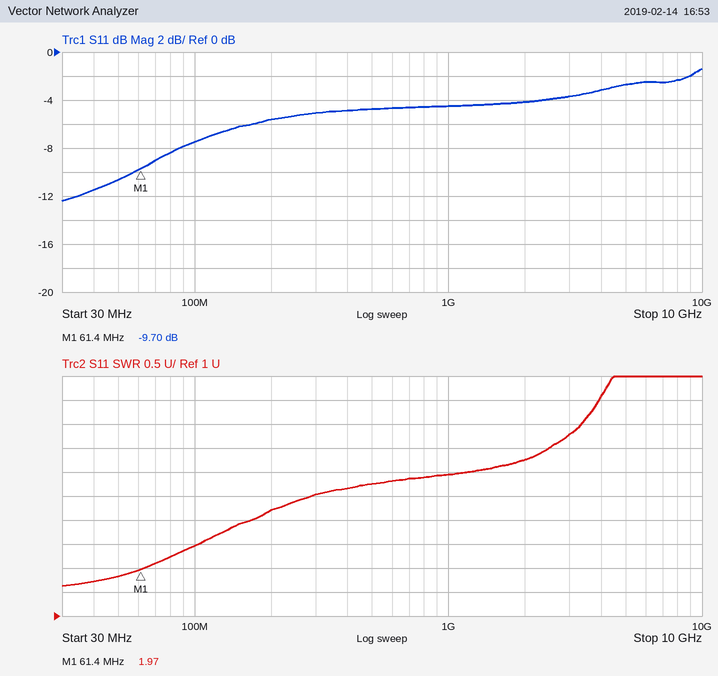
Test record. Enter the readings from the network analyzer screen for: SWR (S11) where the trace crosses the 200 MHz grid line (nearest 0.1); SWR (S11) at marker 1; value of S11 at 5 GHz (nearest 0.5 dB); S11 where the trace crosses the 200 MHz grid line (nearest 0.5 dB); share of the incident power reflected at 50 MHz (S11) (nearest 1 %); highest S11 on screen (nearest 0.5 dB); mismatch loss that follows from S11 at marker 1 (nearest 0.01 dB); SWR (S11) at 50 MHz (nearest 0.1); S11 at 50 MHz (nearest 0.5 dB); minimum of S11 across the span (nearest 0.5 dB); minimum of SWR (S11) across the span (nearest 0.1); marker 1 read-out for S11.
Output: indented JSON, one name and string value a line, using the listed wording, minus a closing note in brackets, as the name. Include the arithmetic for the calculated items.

{
  "SWR (S11) where the trace crosses the 200 MHz grid line": "3.2",
  "SWR (S11) at marker 1": "1.97",
  "value of S11 at 5 GHz": "-2.5 dB",
  "S11 where the trace crosses the 200 MHz grid line": "-5.5 dB",
  "share of the incident power reflected at 50 MHz (S11)": "10^(-10.5/10) ≈ 9 %",
  "highest S11 on screen": "-1.5 dB",
  "mismatch loss that follows from S11 at marker 1": "−10 log10(1 − 10^(-9.7/10)) ≈ 0.49 dB",
  "SWR (S11) at 50 MHz": "1.8",
  "S11 at 50 MHz": "-10.5 dB",
  "minimum of S11 across the span": "-12.5 dB",
  "minimum of SWR (S11) across the span": "1.6",
  "marker 1 read-out for S11": "-9.70 dB"
}
